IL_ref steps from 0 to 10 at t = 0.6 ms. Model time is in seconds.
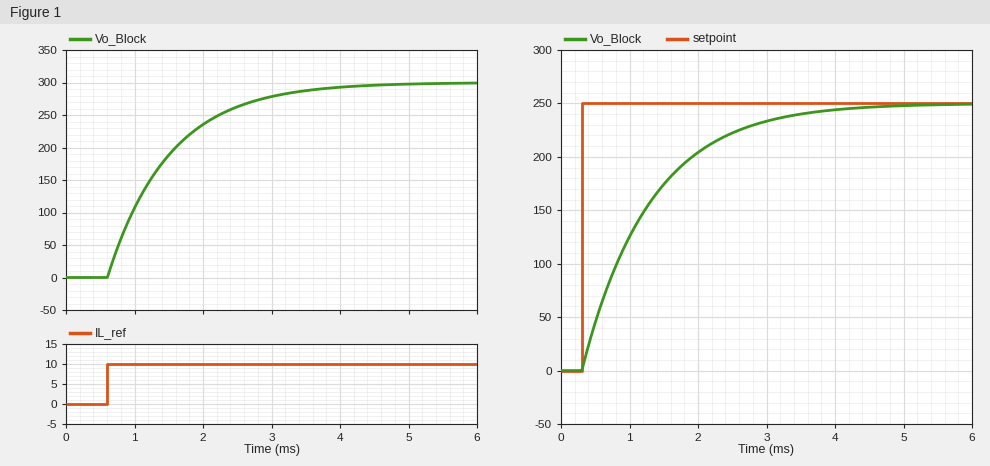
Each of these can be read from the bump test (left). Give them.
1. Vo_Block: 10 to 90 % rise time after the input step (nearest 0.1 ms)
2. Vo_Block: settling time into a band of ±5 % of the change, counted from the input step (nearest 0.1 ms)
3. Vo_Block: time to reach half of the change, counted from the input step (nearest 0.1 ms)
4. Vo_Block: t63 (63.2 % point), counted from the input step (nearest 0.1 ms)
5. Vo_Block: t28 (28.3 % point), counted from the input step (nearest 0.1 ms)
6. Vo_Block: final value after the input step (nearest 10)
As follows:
2.0 ms
2.7 ms
0.6 ms
0.9 ms
0.3 ms
300
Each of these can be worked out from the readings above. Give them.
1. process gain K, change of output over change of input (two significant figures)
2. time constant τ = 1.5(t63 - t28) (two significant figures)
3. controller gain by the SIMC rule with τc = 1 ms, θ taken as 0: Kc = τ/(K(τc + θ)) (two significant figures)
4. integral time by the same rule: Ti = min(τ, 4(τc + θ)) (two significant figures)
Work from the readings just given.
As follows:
30
0.90 ms
0.030
0.90 ms
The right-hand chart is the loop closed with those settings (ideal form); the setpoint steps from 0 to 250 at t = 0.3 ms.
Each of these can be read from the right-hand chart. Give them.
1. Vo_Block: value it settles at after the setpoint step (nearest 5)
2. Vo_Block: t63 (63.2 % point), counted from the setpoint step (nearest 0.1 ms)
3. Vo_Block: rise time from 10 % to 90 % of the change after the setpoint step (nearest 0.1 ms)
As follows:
250
1.0 ms
2.2 ms
